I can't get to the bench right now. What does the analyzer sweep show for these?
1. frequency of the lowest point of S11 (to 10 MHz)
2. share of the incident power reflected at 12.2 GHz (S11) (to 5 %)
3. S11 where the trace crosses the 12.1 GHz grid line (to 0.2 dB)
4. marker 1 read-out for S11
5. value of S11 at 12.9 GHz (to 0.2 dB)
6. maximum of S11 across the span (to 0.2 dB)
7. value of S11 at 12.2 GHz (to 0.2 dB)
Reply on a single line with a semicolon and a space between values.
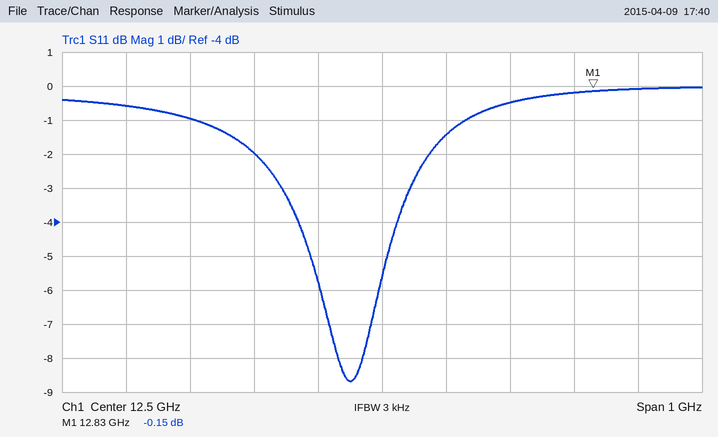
12.45 GHz; 80 %; -0.6 dB; -0.15 dB; 0.0 dB; 0.0 dB; -1.0 dB
